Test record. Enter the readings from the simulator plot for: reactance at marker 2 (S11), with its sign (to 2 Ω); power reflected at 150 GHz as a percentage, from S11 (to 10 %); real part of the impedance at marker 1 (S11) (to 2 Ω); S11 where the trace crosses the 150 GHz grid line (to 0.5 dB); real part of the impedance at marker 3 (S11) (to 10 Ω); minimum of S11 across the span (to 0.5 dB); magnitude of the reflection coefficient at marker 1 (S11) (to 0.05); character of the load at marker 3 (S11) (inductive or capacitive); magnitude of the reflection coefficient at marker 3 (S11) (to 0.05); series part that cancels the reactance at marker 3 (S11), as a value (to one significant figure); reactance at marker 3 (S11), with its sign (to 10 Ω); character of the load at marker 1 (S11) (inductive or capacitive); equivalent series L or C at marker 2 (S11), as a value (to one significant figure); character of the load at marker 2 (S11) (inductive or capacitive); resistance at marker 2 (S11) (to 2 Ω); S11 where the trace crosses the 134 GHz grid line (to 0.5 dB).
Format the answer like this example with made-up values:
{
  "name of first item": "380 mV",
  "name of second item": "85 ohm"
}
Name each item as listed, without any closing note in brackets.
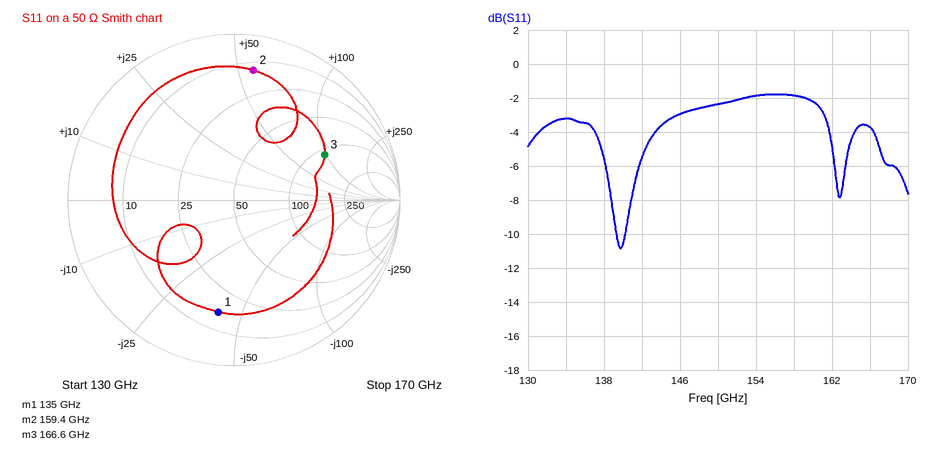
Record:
{
  "reactance at marker 2 (S11), with its sign": "+56 Ω",
  "power reflected at 150 GHz as a percentage, from S11": "60 %",
  "real part of the impedance at marker 1 (S11)": "16 Ω",
  "S11 where the trace crosses the 150 GHz grid line": "-2.5 dB",
  "real part of the impedance at marker 3 (S11)": "110 Ω",
  "minimum of S11 across the span": "-11.0 dB",
  "magnitude of the reflection coefficient at marker 1 (S11)": "0.70",
  "character of the load at marker 3 (S11)": "inductive",
  "magnitude of the reflection coefficient at marker 3 (S11)": "0.60",
  "series part that cancels the reactance at marker 3 (S11), as a value": "10 fF",
  "reactance at marker 3 (S11), with its sign": "+100 Ω",
  "character of the load at marker 1 (S11)": "capacitive",
  "equivalent series L or C at marker 2 (S11), as a value": "60 pH",
  "character of the load at marker 2 (S11)": "inductive",
  "resistance at marker 2 (S11)": "14 Ω",
  "S11 where the trace crosses the 134 GHz grid line": "-3.0 dB"
}
